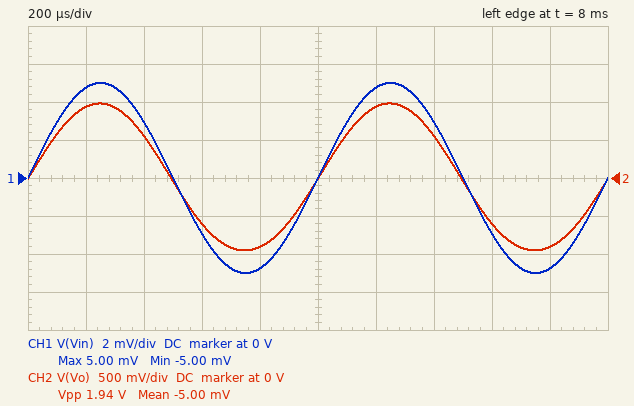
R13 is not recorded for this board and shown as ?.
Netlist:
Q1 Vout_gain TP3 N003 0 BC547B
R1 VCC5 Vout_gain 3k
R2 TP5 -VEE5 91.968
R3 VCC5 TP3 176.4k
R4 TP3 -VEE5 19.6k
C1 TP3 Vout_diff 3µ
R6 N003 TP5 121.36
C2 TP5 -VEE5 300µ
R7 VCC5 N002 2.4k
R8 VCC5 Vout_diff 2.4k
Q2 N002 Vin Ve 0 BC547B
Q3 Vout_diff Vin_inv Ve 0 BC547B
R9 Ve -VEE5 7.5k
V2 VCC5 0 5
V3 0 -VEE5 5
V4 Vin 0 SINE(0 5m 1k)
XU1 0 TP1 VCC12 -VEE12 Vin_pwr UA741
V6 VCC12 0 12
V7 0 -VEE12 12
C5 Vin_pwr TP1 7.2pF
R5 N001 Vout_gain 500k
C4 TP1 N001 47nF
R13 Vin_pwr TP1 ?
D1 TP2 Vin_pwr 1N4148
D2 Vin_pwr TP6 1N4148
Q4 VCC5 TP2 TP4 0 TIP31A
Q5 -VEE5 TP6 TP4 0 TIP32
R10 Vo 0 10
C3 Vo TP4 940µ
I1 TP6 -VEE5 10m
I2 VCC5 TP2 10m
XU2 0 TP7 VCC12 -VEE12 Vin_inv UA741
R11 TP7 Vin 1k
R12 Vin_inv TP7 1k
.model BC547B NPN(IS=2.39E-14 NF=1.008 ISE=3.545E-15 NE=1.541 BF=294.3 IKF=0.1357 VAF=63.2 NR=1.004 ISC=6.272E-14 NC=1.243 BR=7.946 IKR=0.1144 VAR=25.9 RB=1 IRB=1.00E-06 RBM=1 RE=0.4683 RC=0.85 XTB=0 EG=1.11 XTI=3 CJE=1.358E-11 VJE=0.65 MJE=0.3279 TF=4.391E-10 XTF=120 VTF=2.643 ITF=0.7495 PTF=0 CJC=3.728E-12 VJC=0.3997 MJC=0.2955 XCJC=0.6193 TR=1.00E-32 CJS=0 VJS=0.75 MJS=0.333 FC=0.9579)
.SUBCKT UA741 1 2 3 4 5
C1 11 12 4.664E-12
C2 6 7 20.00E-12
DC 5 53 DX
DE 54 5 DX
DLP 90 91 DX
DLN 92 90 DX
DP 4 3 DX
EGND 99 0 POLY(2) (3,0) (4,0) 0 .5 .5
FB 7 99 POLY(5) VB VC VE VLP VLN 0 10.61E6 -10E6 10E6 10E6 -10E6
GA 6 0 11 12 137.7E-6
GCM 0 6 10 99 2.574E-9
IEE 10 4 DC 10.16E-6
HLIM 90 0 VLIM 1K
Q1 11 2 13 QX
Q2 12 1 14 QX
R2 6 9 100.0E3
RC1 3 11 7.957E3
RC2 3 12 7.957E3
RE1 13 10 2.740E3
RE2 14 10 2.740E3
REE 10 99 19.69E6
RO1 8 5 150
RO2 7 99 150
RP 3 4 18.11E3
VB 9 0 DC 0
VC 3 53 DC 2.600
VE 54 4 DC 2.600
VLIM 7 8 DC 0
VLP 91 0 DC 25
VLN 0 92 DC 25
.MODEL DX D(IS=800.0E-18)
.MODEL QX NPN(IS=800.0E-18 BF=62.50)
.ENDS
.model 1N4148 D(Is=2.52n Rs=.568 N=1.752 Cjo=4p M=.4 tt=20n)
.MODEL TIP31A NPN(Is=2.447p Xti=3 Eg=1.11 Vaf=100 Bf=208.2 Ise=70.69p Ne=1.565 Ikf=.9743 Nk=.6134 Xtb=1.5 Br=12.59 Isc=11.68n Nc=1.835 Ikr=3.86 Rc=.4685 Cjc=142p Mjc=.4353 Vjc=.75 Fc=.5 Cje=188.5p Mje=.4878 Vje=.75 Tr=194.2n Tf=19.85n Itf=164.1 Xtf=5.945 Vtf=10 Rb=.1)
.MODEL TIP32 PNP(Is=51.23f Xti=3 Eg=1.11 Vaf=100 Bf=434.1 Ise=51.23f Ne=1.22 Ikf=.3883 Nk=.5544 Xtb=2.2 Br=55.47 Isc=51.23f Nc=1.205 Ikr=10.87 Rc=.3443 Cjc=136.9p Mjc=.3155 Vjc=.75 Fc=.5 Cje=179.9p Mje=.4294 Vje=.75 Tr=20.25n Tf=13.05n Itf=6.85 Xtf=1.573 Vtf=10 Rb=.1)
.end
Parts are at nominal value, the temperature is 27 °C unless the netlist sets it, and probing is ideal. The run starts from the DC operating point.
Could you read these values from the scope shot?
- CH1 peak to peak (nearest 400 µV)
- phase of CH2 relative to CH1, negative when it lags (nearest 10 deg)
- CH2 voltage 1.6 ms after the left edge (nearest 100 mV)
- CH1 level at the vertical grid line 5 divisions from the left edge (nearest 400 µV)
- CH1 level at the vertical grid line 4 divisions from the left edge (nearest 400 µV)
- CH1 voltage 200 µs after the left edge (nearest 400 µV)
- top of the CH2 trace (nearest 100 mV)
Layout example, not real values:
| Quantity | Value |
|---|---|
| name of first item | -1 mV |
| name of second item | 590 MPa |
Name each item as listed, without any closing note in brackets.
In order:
| Quantity | Value |
|---|---|
| CH1 peak to peak | 10.0 mV |
| phase of CH2 relative to CH1, negative when it lags | 0 deg |
| CH2 voltage 1.6 ms after the left edge | -600 mV |
| CH1 level at the vertical grid line 5 divisions from the left edge | 0 V |
| CH1 level at the vertical grid line 4 divisions from the left edge | -4.8 mV |
| CH1 voltage 200 µs after the left edge | 4.8 mV |
| top of the CH2 trace | 1.0 V |
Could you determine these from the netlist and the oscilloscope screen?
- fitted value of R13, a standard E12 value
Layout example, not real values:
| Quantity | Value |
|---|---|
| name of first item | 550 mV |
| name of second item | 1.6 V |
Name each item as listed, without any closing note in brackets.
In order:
| Quantity | Value |
|---|---|
| fitted value of R13, a standard E12 value | 220 kΩ |
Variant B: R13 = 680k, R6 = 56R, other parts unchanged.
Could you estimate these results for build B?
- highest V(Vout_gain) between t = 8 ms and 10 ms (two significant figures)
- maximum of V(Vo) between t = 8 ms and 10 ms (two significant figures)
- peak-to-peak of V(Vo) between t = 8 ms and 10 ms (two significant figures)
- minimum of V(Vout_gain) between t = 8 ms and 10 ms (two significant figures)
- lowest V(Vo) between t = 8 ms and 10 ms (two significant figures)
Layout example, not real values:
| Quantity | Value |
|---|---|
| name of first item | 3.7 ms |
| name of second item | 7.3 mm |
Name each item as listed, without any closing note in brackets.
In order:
| Quantity | Value |
|---|---|
| highest V(Vout_gain) between t = 8 ms and 10 ms | 3.7 V |
| maximum of V(Vo) between t = 8 ms and 10 ms | 4.6 V |
| peak-to-peak of V(Vo) between t = 8 ms and 10 ms | 9.5 V |
| minimum of V(Vout_gain) between t = 8 ms and 10 ms | -4.4 V |
| lowest V(Vo) between t = 8 ms and 10 ms | -4.9 V |
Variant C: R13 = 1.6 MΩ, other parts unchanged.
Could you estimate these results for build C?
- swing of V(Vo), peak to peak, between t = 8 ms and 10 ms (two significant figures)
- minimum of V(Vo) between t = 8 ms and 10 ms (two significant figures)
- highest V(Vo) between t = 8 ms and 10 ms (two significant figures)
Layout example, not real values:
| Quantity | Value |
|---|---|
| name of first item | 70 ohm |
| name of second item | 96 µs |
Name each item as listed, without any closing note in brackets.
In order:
| Quantity | Value |
|---|---|
| swing of V(Vo), peak to peak, between t = 8 ms and 10 ms | 9.6 V |
| minimum of V(Vo) between t = 8 ms and 10 ms | -4.9 V |
| highest V(Vo) between t = 8 ms and 10 ms | 4.6 V |
